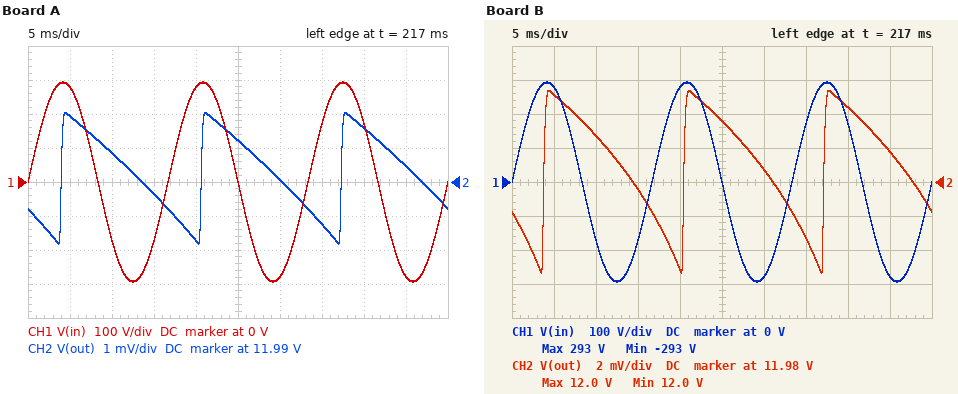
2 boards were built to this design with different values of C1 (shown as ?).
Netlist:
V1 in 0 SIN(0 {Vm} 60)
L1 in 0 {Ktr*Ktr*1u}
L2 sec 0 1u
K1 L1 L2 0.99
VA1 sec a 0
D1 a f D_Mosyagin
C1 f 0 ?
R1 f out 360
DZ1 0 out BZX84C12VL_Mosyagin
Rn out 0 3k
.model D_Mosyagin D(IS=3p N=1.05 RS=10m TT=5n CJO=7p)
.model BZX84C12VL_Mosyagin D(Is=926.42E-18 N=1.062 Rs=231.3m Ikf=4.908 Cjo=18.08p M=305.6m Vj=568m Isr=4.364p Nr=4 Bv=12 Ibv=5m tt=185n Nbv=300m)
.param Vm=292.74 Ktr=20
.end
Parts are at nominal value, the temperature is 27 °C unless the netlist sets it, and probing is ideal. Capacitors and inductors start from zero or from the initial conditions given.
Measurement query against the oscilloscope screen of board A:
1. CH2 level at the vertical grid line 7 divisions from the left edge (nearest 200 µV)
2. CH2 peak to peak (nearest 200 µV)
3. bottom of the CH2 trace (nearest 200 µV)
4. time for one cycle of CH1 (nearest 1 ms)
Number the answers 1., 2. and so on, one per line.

1. 11.9858 V
2. 3.8 mV
3. 11.9852 V
4. 17 ms
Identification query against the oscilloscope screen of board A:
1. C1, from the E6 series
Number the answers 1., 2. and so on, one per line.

1. 470 µF
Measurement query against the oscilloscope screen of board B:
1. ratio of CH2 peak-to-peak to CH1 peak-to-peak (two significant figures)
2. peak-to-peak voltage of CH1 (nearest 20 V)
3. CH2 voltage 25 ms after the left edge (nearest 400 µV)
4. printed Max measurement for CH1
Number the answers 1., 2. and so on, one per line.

1. 0.000018
2. 580 V
3. 11.9876 V
4. 293 V
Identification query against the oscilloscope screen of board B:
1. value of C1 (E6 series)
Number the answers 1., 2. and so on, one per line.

1. 220 µF
